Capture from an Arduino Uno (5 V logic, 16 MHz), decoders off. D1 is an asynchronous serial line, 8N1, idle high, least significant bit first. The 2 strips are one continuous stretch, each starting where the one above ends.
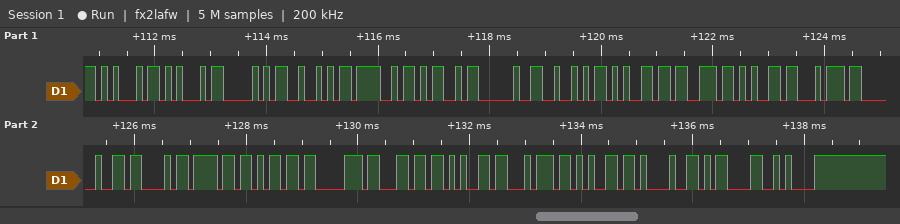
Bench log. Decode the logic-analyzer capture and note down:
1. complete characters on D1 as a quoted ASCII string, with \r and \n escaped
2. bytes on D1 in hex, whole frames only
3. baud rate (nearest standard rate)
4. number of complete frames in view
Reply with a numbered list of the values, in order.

1. "EEPROM Reset Complete!\r\n"
2. 45 45 50 52 4F 4D 20 52 65 73 65 74 20 43 6F 6D 70 6C 65 74 65 21 0D 0A
3. 9600 baud
4. 24
